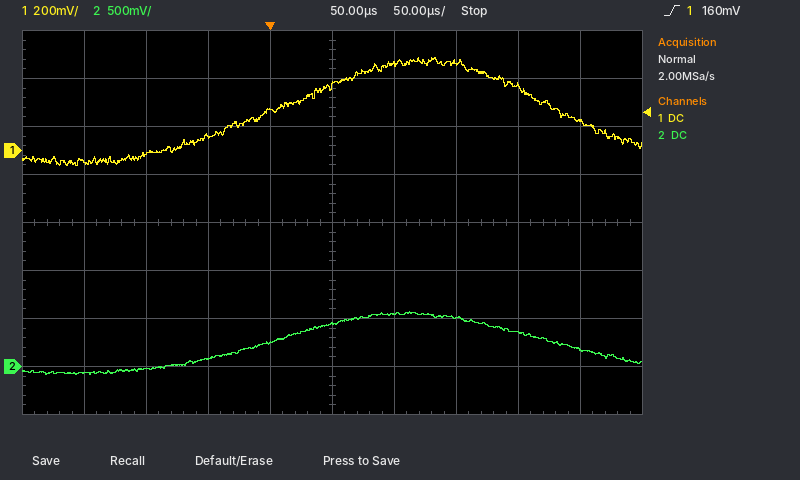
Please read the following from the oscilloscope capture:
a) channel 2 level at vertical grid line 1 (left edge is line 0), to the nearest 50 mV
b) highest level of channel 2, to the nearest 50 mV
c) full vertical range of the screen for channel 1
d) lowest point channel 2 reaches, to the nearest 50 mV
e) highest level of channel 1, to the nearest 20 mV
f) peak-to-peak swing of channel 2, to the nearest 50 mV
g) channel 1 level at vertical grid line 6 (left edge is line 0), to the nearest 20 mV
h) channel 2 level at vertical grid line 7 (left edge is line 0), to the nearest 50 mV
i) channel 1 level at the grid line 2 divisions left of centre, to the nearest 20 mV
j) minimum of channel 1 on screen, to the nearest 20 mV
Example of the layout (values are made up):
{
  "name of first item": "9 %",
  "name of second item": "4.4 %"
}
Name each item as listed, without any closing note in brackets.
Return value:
{
  "channel 2 level at vertical grid line 1 (left edge is line 0), to the nearest 50 mV": "-50 mV",
  "highest level of channel 2, to the nearest 50 mV": "550 mV",
  "full vertical range of the screen for channel 1": "1.6 V",
  "lowest point channel 2 reaches, to the nearest 50 mV": "-100 mV",
  "highest level of channel 1, to the nearest 20 mV": "380 mV",
  "peak-to-peak swing of channel 2, to the nearest 50 mV": "650 mV",
  "channel 1 level at vertical grid line 6 (left edge is line 0), to the nearest 20 mV": "360 mV",
  "channel 2 level at vertical grid line 7 (left edge is line 0), to the nearest 50 mV": "500 mV",
  "channel 1 level at the grid line 2 divisions left of centre, to the nearest 20 mV": "60 mV",
  "minimum of channel 1 on screen, to the nearest 20 mV": "-60 mV"
}
